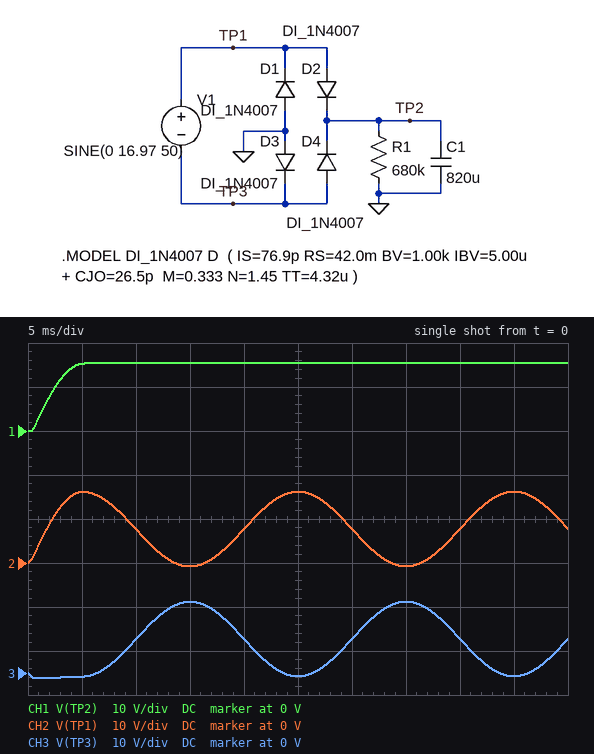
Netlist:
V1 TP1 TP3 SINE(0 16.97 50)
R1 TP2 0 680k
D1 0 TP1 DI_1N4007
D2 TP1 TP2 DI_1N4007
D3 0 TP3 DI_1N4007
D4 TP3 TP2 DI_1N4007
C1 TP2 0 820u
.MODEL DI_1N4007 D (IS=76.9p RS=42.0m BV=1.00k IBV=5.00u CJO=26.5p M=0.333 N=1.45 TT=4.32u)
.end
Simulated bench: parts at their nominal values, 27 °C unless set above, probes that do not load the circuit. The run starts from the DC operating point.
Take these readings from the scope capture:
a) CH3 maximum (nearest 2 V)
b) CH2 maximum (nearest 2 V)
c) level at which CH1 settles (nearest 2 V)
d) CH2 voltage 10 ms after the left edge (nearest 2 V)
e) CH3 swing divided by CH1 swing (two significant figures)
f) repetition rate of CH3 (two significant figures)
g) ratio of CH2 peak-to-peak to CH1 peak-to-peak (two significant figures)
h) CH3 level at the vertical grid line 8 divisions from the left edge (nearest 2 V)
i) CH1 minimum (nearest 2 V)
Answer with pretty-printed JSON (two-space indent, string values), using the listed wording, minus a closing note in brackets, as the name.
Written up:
{
  "CH3 maximum": "16 V",
  "CH2 maximum": "16 V",
  "level at which CH1 settles": "16 V",
  "CH2 voltage 10 ms after the left edge": "8 V",
  "CH3 swing divided by CH1 swing": "1.1",
  "repetition rate of CH3": "50 Hz",
  "ratio of CH2 peak-to-peak to CH1 peak-to-peak": "1.1",
  "CH3 level at the vertical grid line 8 divisions from the left edge": "8 V",
  "CH1 minimum": "0 V"
}
